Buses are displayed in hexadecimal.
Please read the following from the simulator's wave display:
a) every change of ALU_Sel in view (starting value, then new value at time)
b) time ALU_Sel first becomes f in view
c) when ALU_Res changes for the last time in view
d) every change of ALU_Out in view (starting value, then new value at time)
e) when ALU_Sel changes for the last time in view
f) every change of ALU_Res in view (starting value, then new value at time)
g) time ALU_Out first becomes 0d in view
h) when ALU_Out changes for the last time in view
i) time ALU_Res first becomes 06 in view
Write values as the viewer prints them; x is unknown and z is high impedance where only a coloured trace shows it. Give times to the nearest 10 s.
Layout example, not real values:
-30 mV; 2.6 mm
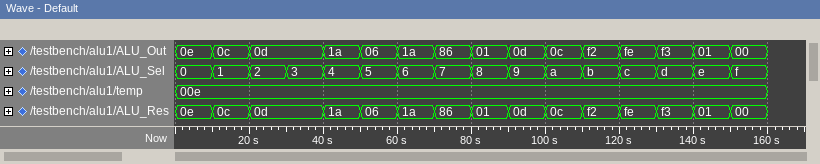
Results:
0, 1 at 10 s, 2 at 20 s, 3 at 30 s, 4 at 40 s, 5 at 50 s, 6 at 60 s, 7 at 70 s, 8 at 80 s, 9 at 90 s, a at 100 s, b at 110 s, c at 120 s, d at 130 s, e at 140 s, f at 150 s; 150 s; 150 s; 0e, 0c at 10 s, 0d at 20 s, 1a at 40 s, 06 at 50 s, 1a at 60 s, 86 at 70 s, 01 at 80 s, 0d at 90 s, 0c at 100 s, f2 at 110 s, fe at 120 s, f3 at 130 s, 01 at 140 s, 00 at 150 s; 150 s; 0e, 0c at 10 s, 0d at 20 s, 1a at 40 s, 06 at 50 s, 1a at 60 s, 86 at 70 s, 01 at 80 s, 0d at 90 s, 0c at 100 s, f2 at 110 s, fe at 120 s, f3 at 130 s, 01 at 140 s, 00 at 150 s; 20 s; 150 s; 50 s
